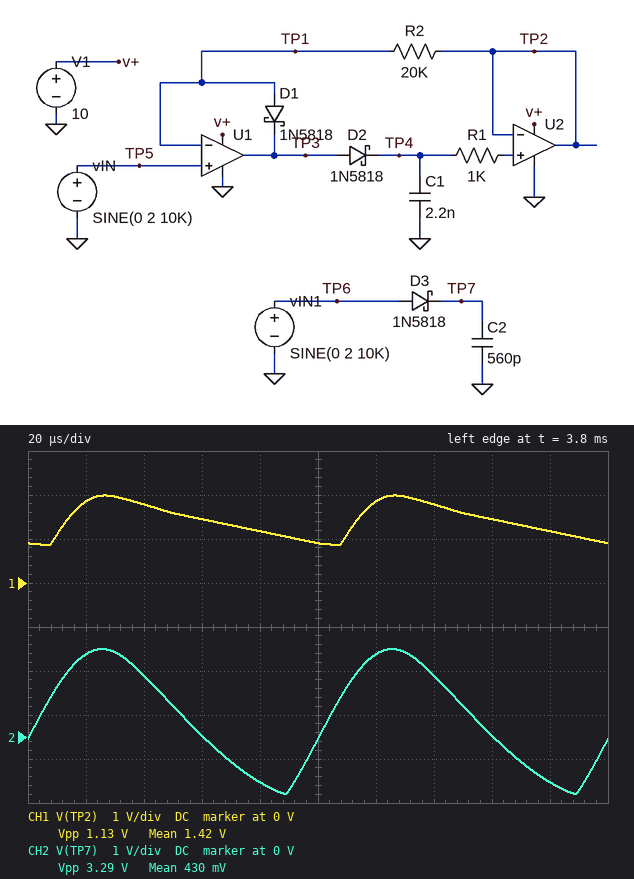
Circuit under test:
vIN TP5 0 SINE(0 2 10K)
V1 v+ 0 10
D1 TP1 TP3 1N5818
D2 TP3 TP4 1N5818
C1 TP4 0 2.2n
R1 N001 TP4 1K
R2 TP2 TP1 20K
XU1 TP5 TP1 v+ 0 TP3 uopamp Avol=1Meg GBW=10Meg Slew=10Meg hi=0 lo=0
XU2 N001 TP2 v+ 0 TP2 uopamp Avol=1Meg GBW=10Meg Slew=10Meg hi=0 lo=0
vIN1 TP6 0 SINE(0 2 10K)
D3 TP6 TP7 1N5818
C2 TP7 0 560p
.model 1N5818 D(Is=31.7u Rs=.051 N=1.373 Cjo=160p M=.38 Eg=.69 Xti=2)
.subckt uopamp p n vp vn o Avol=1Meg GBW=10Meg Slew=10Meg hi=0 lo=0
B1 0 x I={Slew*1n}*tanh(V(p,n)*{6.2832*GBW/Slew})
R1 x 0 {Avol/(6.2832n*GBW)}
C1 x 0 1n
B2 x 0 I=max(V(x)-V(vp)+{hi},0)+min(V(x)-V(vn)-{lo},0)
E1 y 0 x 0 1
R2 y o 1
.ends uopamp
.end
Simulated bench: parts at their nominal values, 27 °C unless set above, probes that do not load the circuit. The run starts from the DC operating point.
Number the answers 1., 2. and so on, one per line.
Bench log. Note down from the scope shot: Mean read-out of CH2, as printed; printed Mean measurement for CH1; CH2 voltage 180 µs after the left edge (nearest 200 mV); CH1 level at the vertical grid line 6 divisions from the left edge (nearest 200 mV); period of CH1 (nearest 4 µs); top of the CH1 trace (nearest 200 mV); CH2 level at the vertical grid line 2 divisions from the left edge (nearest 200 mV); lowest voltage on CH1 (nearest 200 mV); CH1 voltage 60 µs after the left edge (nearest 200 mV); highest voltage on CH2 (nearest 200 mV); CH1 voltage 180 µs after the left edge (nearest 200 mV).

1. 430 mV
2. 1.42 V
3. -1.0 V
4. 1.8 V
5. 100 µs
6. 2.0 V
7. 1.4 V
8. 800 mV
9. 1.4 V
10. 2.0 V
11. 1.2 V
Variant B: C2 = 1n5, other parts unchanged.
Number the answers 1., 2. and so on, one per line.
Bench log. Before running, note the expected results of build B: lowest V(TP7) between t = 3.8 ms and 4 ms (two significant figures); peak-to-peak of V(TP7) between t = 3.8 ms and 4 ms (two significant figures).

1. 420 mV
2. 1.6 V
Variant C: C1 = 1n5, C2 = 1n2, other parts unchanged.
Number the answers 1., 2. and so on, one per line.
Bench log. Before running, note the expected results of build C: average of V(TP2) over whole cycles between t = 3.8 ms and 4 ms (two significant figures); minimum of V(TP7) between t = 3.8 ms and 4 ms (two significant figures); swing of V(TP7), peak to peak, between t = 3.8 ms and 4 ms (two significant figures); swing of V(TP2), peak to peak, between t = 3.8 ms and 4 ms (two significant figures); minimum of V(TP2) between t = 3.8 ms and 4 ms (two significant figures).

1. 1.2 V
2. 100 mV
3. 1.9 V
4. 1.6 V
5. 420 mV
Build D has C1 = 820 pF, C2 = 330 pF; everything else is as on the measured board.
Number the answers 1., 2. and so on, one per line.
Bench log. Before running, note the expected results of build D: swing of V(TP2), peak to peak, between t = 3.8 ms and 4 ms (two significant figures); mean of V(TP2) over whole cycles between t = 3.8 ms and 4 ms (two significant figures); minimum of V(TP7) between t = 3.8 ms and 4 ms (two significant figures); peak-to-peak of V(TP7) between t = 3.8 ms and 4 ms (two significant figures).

1. 2.0 V
2. 870 mV
3. -2.0 V
4. 4.0 V
